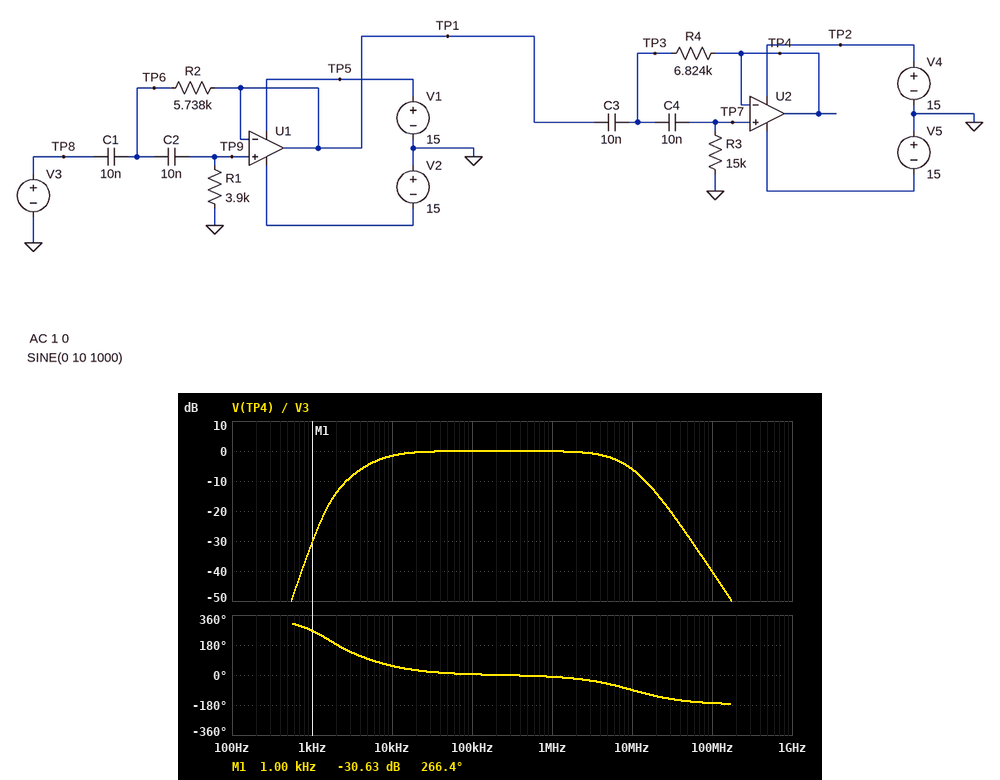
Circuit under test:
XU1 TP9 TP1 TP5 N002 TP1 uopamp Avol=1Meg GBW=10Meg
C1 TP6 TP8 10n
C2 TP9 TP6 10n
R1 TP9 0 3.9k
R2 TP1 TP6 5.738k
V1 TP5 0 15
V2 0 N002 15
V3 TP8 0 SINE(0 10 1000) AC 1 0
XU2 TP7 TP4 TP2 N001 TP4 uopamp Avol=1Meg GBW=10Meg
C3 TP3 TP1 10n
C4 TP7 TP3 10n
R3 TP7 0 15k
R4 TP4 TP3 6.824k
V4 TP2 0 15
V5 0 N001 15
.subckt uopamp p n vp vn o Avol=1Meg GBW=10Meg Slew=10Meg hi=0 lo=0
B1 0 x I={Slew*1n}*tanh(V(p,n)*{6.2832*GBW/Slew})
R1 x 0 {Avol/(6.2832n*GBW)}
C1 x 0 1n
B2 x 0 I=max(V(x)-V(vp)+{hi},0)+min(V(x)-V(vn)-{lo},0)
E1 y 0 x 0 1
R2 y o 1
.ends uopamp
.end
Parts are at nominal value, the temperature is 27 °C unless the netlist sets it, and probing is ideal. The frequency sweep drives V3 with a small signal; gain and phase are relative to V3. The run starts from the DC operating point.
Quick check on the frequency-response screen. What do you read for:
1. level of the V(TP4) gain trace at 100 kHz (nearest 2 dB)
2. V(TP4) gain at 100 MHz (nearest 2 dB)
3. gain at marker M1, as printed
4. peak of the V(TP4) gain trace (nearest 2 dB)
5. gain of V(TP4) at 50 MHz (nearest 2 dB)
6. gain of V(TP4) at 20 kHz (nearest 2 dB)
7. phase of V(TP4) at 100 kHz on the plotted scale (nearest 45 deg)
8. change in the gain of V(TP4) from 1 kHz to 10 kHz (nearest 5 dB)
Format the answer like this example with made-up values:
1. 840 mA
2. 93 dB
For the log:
1. 0 dB
2. -40 dB
3. -30.63 dB
4. 0 dB
5. -28 dB
6. 0 dB
7. 0 deg
8. 30 dB
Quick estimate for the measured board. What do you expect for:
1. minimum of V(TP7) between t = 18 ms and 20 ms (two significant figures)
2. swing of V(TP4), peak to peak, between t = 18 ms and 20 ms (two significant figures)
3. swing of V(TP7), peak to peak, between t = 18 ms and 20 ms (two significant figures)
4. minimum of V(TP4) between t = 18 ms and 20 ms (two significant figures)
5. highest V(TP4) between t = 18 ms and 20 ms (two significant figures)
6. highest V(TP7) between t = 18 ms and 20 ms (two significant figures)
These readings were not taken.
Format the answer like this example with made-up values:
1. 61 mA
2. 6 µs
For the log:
1. -290 mV
2. 590 mV
3. 590 mV
4. -290 mV
5. 290 mV
6. 290 mV
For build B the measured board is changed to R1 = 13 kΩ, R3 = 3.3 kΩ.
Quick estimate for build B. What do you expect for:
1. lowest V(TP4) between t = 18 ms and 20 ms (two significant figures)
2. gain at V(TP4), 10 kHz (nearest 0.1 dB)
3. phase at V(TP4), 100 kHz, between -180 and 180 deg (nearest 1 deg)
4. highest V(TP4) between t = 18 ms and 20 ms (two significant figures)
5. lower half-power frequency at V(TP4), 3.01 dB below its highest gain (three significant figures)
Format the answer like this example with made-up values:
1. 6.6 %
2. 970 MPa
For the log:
1. -210 mV
2. -2.3 dB
3. 6 deg
4. 210 mV
5. 8.41 kHz
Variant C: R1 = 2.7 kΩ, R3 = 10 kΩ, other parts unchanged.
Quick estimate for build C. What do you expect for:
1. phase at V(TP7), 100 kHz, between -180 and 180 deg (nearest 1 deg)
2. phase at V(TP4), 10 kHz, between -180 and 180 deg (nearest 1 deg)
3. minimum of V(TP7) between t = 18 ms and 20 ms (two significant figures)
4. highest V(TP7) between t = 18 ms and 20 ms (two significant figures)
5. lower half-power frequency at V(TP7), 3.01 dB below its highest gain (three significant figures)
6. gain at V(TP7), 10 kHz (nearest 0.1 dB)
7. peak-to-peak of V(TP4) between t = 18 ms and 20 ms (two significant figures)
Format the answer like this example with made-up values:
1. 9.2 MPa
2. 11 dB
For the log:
1. 8 deg
2. 73 deg
3. -120 mV
4. 120 mV
5. 10.7 kHz
6. -3.3 dB
7. 250 mV
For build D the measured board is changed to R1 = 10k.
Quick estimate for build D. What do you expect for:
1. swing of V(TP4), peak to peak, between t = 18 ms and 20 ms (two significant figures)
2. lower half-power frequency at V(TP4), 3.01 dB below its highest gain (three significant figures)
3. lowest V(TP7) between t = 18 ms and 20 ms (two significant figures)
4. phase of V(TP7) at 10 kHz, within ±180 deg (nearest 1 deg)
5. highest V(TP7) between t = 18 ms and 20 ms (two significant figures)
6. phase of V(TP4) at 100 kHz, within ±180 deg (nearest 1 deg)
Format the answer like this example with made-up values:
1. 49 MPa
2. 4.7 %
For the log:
1. 1.7 V
2. 2.40 kHz
3. -830 mV
4. 31 deg
5. 830 mV
6. 2 deg
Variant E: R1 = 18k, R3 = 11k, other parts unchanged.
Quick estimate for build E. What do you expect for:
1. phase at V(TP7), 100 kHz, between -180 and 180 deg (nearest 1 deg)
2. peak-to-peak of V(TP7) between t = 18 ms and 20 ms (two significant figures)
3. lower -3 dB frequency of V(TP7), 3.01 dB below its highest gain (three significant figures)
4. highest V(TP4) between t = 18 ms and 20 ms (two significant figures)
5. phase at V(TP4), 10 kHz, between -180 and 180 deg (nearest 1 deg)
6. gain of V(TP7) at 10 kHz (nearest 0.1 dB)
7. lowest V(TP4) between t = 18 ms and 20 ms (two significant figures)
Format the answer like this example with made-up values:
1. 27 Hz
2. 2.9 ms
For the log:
1. 2 deg
2. 2.3 V
3. 1.99 kHz
4. 1.2 V
5. 27 deg
6. 0 dB
7. -1.2 V
